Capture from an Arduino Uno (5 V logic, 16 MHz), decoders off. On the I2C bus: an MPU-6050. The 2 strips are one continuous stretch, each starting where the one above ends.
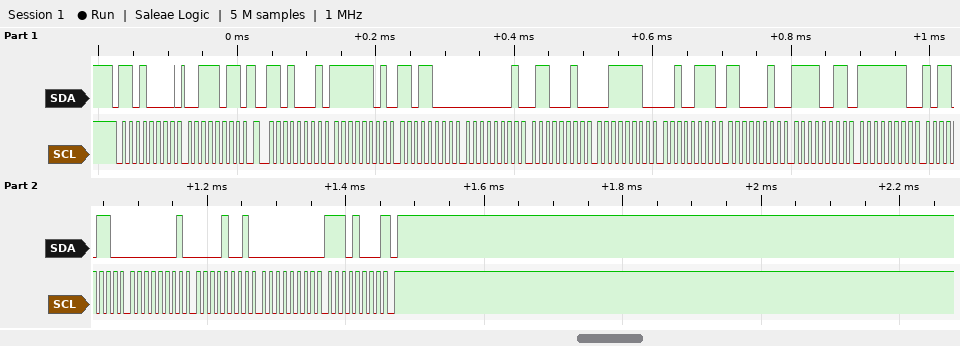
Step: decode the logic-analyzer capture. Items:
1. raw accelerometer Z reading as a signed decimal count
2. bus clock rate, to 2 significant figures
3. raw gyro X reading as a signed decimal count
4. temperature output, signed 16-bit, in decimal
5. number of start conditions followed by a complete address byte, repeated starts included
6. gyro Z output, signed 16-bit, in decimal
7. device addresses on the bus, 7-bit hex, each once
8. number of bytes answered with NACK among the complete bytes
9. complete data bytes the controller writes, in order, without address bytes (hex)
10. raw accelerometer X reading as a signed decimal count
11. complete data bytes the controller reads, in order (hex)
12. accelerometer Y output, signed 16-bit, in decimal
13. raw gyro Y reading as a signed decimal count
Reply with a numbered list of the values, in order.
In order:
1. 15911
2. 100 kHz
3. -330
4. -15629
5. 2
6. 232
7. 0x68
8. 1
9. 3B
10. -552
11. FD D8 01 62 3E 27 C2 F3 FE B6 01 09 00 E8
12. 354
13. 265
